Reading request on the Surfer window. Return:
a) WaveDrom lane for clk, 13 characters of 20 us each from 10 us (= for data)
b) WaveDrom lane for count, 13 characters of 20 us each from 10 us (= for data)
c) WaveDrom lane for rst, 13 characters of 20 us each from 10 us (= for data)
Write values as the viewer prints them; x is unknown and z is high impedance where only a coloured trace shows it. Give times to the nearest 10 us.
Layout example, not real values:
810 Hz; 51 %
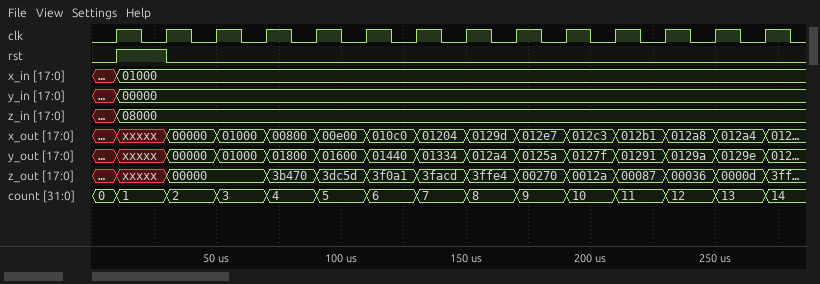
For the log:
{name: 'clk', wave: 'p............'}; {name: 'count', wave: '=============', data: '1 2 3 4 5 6 7 8 9 10 11 12 13'}; {name: 'rst', wave: '10...........'}
